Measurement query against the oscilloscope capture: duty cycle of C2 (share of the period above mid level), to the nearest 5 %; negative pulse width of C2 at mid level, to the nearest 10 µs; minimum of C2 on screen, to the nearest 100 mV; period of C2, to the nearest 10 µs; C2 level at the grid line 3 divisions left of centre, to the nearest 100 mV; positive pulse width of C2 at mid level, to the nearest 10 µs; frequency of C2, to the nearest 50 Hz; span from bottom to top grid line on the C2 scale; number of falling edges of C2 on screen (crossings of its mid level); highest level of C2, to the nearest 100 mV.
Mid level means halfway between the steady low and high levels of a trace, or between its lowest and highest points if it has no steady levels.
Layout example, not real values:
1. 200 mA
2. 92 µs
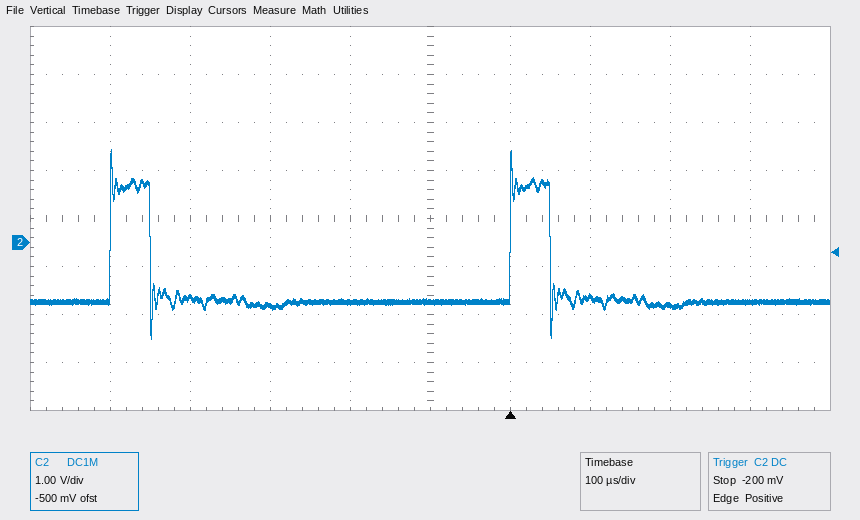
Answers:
1. 10 %
2. 450 µs
3. -2.0 V
4. 500 µs
5. -1.2 V
6. 50 µs
7. 2.00 kHz
8. 8 V
9. 2
10. 1.9 V
